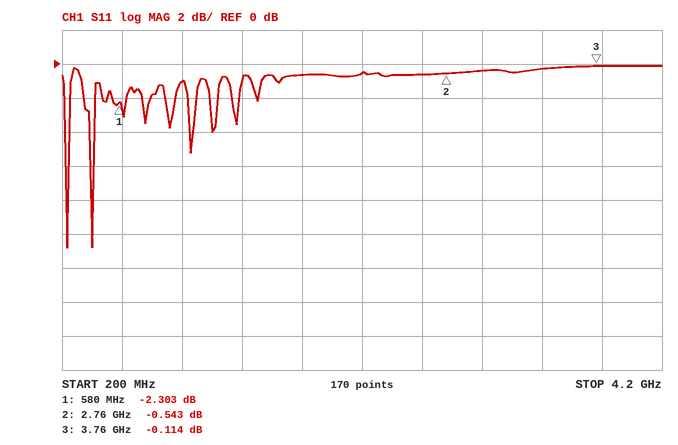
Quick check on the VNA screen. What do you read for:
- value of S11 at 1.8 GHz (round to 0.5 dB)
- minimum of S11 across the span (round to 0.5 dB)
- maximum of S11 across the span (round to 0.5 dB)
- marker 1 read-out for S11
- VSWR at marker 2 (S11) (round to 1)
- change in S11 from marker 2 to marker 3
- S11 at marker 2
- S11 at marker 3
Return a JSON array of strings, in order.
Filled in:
["-0.5 dB", "-11.0 dB", "0.0 dB", "-2.303 dB", "32", "0.429 dB", "-0.543 dB", "-0.114 dB"]
